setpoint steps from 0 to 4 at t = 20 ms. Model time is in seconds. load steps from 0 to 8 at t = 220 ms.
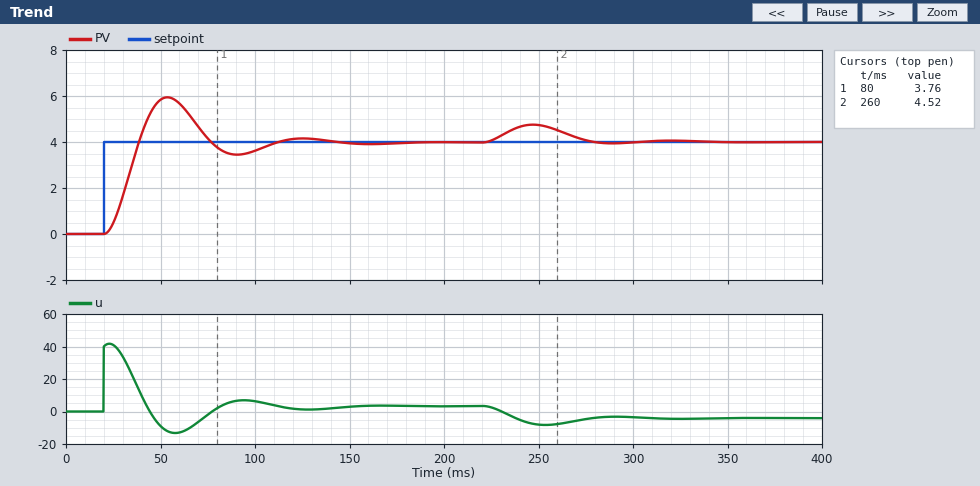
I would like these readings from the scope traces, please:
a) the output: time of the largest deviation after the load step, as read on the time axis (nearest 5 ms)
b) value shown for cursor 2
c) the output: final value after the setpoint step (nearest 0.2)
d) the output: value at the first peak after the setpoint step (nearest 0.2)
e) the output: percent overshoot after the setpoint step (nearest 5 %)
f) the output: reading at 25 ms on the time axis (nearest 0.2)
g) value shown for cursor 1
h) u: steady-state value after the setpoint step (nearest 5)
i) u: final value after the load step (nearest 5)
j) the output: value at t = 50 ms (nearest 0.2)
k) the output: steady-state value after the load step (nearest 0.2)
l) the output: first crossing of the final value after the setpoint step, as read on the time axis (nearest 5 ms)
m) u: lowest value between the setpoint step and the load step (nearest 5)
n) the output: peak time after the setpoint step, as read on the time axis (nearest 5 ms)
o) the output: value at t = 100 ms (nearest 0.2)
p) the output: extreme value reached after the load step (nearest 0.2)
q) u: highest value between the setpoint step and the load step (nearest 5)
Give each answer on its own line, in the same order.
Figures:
245 ms
4.52
4.0
6.0
50 %
0.4
3.76
5
-5
5.8
4.0
40 ms
-15
55 ms
3.6
4.8
40
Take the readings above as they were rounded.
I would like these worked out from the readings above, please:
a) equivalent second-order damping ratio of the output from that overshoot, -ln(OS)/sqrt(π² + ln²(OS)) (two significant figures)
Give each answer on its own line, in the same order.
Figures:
0.22
